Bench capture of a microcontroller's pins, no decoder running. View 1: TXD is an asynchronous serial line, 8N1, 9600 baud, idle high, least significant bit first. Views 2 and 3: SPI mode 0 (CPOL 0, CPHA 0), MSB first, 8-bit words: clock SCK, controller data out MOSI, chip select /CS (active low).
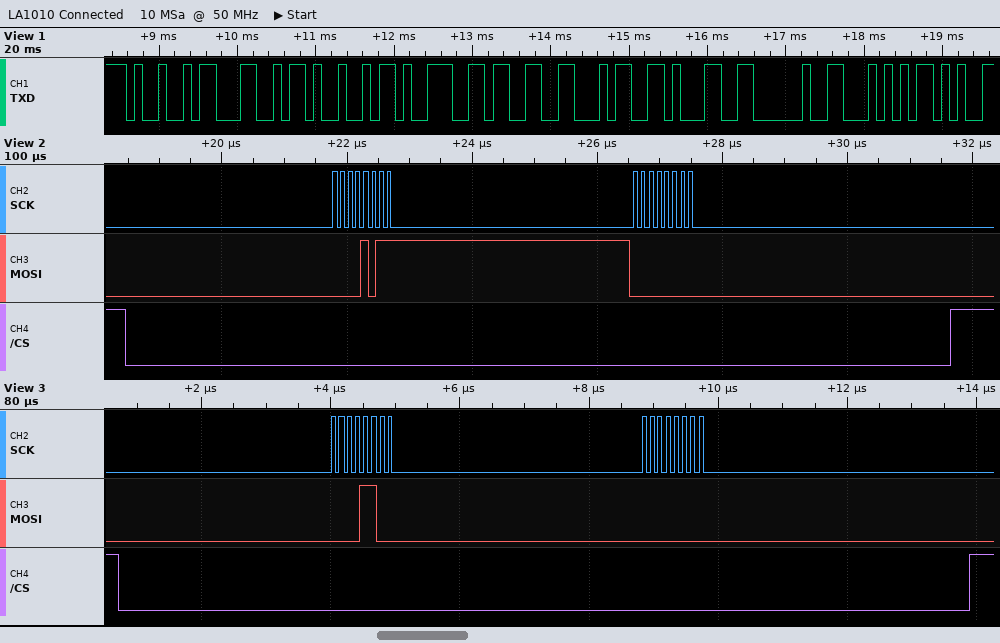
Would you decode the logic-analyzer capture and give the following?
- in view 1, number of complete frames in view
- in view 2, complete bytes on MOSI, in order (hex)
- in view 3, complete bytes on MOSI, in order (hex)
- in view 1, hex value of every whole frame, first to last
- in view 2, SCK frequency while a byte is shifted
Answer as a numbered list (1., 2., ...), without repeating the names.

1. 9
2. 0B 00
3. 0C 00
4. 49 4C 49 39 33 34 31 20 54
5. 8 MHz
